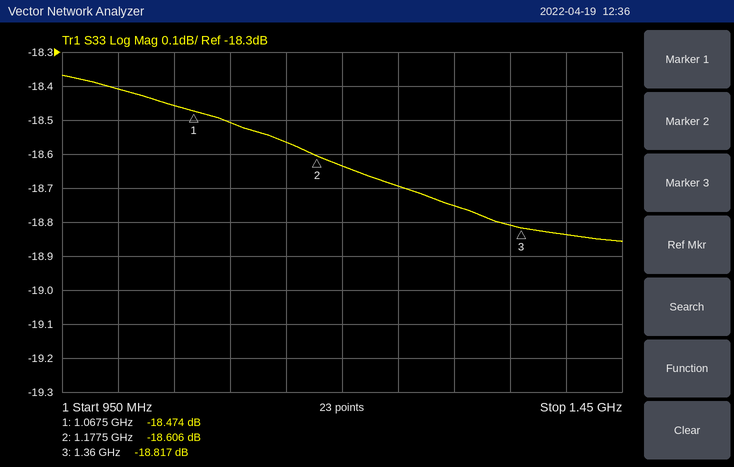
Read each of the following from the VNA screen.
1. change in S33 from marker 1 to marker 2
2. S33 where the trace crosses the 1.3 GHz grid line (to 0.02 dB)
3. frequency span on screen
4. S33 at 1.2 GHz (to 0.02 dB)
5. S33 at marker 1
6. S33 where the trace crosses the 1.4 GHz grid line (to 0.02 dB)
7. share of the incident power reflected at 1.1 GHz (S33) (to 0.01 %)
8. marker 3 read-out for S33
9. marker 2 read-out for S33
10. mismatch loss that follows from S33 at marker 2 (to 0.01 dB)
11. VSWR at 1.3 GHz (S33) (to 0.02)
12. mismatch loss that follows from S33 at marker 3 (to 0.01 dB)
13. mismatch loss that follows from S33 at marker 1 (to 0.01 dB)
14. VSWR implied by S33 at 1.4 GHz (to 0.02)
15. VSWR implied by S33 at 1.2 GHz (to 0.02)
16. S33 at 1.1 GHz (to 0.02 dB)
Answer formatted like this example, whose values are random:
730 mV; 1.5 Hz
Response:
-0.132 dB; -18.76 dB; 500 MHz; -18.64 dB; -18.474 dB; -18.84 dB; 1.41 %; -18.817 dB; -18.606 dB; 0.06 dB; 1.26; 0.06 dB; 0.06 dB; 1.26; 1.26; -18.50 dB
